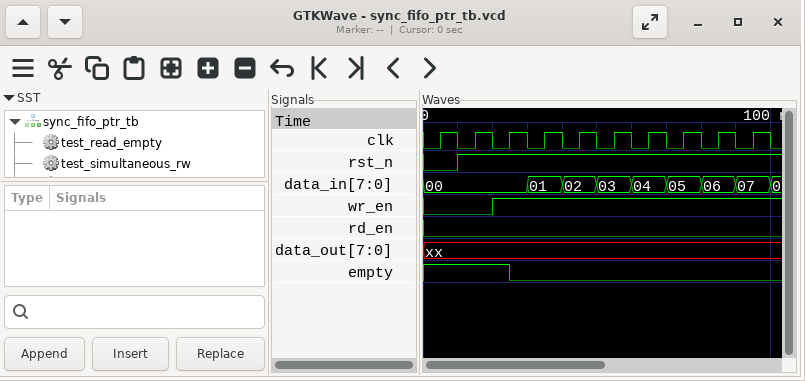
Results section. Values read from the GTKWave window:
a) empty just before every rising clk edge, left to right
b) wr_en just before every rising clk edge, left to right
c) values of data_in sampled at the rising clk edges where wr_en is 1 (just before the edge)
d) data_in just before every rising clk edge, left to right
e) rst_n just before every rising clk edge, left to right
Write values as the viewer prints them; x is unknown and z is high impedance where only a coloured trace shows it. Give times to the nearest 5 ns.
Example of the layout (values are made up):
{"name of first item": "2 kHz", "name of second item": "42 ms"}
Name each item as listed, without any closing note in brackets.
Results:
{"empty just before every rising clk edge, left to right": "1 1 1 0 0 0 0 0 0 0", "wr_en just before every rising clk edge, left to right": "0 0 1 1 1 1 1 1 1 1", "values of data_in sampled at the rising clk edges where wr_en is 1": "00, 01, 02, 03, 04, 05, 06, 07", "data_in just before every rising clk edge, left to right": "00, 00, 00, 01, 02, 03, 04, 05, 06, 07", "rst_n just before every rising clk edge, left to right": "0 1 1 1 1 1 1 1 1 1"}
